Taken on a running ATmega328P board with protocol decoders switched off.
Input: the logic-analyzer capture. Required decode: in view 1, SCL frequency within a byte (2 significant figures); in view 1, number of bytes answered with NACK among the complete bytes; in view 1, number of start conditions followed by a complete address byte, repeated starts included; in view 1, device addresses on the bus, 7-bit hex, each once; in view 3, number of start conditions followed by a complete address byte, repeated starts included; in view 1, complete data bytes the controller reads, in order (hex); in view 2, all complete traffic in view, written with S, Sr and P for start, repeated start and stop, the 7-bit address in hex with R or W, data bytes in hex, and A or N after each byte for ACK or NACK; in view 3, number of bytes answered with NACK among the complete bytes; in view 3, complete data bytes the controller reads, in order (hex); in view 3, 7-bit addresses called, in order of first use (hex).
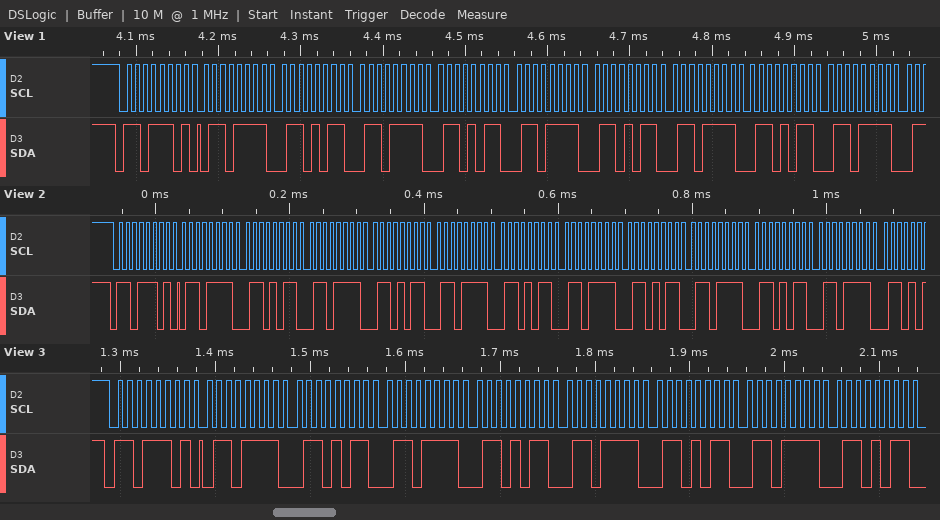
100 kHz
0
1
0x6E
1
6F 6B 6F 6B 6F 6B 6F 6B 6F
S 6ER A 6F A 6B A 6F A 6B A 6F A 6B A 6F A 6B A 6F A 6B A 6F A
0
6F 6B 6F 6B 6F 6B 6F 6B
0x6E
